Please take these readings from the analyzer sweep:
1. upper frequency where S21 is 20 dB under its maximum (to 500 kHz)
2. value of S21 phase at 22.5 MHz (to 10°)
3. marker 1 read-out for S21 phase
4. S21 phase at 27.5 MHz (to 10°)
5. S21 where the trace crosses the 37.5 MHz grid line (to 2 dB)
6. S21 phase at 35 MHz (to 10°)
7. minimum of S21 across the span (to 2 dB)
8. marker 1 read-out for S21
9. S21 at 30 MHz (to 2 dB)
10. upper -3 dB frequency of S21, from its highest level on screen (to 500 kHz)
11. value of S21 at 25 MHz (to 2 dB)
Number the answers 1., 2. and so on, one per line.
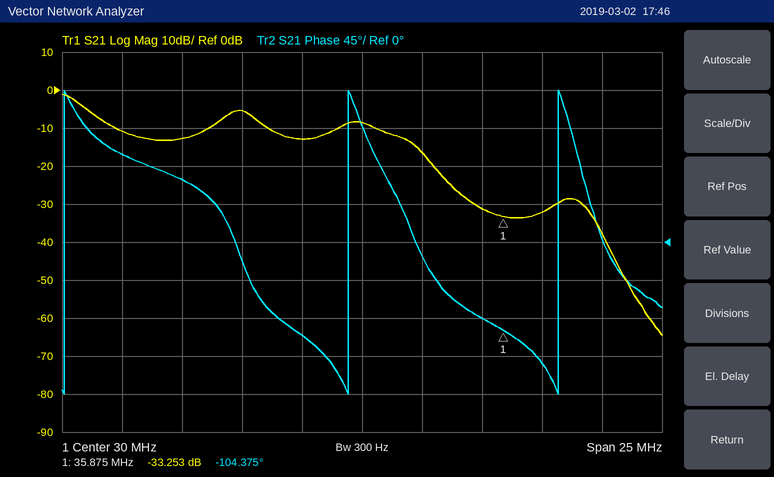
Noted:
1. 33.0 MHz
2. 70°
3. -104.375°
4. -110°
5. -32 dB
6. -90°
7. -64 dB
8. -33.253 dB
9. -8 dB
10. 18.5 MHz
11. -6 dB
